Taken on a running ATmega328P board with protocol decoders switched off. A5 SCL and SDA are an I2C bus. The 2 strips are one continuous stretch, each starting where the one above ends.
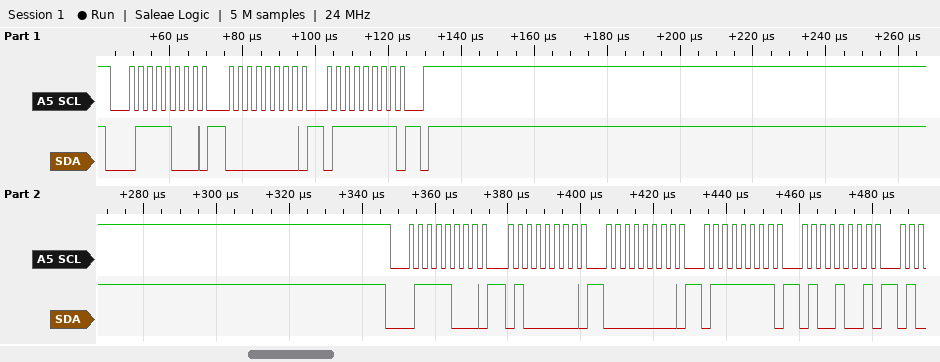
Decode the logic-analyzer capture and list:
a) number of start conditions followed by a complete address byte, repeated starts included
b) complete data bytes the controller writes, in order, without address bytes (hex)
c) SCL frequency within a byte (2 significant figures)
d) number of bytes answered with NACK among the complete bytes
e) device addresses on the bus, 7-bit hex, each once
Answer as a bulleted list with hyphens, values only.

- 2
- 00 7F 40 00 7F 49
- 400 kHz
- 0
- 0x3C
